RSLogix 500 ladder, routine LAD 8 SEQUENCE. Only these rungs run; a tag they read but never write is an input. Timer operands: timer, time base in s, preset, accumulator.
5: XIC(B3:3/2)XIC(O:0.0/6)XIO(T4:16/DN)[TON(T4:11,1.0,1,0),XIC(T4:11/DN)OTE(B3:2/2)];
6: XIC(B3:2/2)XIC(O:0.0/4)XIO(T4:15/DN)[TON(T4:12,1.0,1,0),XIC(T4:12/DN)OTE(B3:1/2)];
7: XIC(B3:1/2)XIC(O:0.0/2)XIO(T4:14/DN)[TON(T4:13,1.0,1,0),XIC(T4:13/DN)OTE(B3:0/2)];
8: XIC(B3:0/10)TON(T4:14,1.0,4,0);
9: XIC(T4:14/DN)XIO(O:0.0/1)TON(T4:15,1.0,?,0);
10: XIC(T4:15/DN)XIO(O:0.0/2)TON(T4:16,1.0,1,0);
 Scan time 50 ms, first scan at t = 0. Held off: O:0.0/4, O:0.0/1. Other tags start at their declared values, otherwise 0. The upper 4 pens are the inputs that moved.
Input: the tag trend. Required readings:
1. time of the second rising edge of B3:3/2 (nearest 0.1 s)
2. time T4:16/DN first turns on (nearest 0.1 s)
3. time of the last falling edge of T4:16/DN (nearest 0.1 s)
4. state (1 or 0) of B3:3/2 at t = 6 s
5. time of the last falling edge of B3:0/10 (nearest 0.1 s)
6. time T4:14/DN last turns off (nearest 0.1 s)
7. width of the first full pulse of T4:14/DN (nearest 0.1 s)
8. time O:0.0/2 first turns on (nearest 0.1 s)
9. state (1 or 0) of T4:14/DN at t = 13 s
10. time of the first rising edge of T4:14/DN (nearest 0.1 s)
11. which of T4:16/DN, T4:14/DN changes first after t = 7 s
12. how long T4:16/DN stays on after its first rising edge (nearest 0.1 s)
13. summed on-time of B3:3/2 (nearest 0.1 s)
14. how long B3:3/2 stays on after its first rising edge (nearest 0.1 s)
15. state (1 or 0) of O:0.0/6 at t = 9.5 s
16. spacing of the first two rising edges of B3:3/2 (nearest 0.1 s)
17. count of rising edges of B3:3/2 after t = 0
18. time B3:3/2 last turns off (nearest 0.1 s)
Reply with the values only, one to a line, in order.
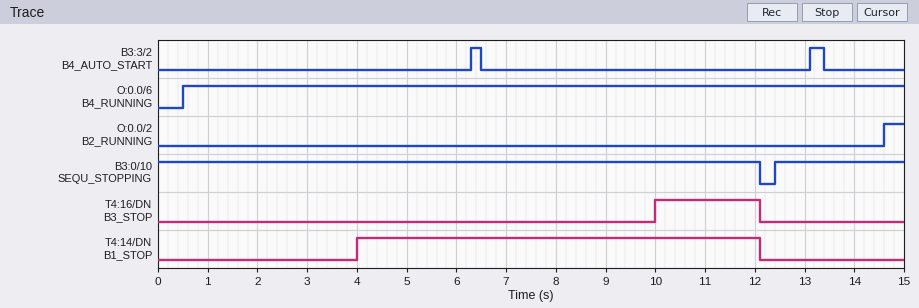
13.1 s
10.0 s
12.1 s
0
12.1 s
12.1 s
8.1 s
14.6 s
0
4.0 s
T4:16/DN
2.1 s
0.5 s
0.2 s
1
6.8 s
2
13.4 s
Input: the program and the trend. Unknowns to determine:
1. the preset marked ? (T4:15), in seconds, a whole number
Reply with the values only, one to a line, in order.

5 s
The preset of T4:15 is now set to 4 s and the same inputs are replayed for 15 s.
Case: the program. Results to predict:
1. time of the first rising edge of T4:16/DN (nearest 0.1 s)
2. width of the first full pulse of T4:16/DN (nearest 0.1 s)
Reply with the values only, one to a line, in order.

9.0 s
3.1 s
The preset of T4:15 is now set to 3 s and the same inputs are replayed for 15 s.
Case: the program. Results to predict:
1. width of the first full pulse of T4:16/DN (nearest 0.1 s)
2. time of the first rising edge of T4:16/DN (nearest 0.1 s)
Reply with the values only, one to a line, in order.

4.1 s
8.0 s
